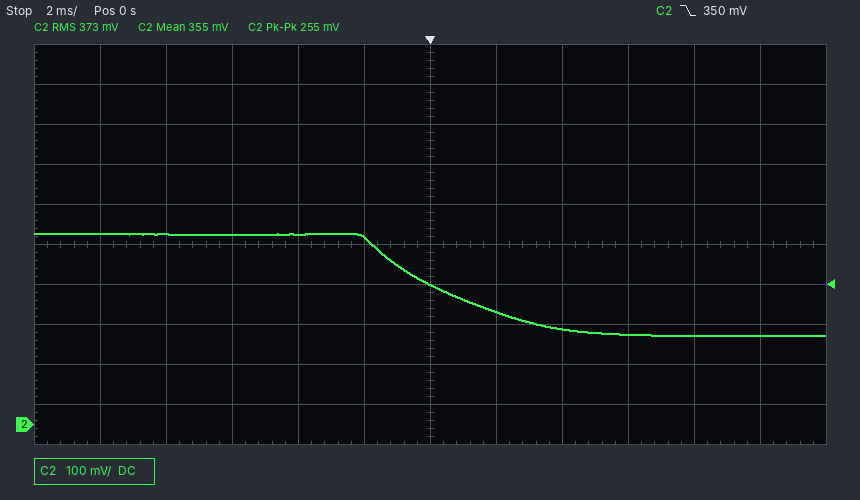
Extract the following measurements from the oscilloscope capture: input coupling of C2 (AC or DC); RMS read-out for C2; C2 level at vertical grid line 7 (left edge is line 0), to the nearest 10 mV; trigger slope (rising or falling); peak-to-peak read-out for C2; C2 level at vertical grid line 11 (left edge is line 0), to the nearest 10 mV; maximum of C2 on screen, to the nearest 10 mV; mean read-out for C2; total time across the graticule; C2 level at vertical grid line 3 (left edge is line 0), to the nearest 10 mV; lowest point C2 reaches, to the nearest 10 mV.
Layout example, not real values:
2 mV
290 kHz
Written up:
DC
373 mV
280 mV
falling
255 mV
220 mV
480 mV
355 mV
24 ms
480 mV
220 mV
